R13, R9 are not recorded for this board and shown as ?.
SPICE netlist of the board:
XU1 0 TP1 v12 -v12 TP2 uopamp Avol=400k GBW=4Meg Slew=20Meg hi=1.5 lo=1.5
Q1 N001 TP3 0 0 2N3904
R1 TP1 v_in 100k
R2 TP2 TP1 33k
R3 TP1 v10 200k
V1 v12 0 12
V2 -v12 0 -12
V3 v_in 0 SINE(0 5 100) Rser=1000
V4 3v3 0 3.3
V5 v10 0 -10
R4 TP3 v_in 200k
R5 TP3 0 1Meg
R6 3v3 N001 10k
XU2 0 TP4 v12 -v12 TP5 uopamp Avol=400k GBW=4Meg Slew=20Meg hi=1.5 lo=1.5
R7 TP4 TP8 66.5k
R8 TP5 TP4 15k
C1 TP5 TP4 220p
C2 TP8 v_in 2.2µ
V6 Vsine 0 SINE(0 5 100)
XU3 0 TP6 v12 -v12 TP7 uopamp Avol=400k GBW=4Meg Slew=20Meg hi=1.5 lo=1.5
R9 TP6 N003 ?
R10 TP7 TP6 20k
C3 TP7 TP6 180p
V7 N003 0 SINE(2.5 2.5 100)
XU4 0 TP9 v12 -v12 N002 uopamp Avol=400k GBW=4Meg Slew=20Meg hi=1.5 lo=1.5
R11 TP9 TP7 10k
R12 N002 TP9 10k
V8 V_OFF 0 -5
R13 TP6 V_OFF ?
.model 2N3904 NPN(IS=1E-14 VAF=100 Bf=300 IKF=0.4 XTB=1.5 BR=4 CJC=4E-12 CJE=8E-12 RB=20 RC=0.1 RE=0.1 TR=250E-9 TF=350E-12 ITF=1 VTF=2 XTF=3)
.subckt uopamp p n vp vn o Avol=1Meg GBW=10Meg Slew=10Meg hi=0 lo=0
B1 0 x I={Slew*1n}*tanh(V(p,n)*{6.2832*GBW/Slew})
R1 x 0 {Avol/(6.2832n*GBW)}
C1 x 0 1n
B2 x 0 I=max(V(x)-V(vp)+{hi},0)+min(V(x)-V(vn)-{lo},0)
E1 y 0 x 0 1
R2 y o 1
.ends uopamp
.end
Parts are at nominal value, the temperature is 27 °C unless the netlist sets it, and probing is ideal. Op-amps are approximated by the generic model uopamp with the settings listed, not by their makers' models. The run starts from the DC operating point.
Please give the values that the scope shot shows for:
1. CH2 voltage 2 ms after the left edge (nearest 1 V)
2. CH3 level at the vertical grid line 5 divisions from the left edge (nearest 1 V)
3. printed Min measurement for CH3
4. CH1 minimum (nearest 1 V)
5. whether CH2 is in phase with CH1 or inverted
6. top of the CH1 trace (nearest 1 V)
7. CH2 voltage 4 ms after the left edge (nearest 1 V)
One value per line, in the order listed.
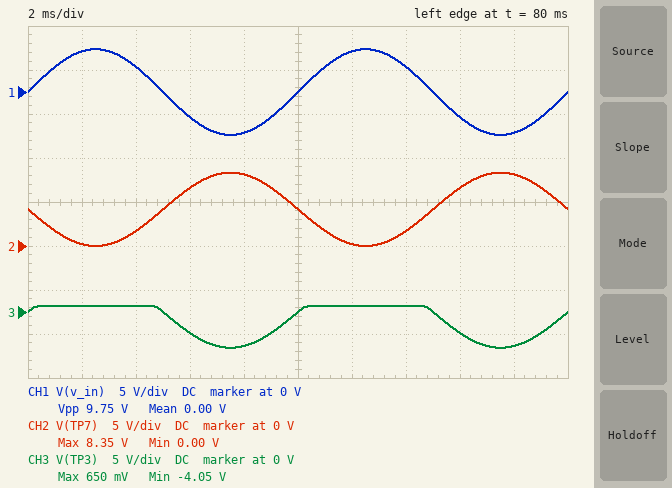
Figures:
0 V
0 V
-4.05 V
-5 V
inverted
5 V
2 V
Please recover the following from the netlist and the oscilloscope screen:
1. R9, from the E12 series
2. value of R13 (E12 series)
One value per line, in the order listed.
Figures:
12 kΩ
12 kΩ
